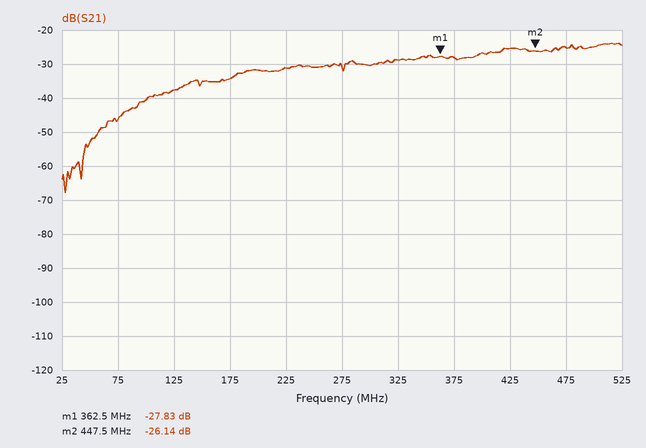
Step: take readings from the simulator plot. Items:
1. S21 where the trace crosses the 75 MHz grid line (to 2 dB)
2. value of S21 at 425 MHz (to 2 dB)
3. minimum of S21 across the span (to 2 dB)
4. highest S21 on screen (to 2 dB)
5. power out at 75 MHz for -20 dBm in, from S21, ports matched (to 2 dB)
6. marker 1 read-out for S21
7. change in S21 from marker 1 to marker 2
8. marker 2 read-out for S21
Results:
-46 dB
-26 dB
-68 dB
-24 dB
-66 dBm
-27.83 dB
1.69 dB
-26.14 dB
